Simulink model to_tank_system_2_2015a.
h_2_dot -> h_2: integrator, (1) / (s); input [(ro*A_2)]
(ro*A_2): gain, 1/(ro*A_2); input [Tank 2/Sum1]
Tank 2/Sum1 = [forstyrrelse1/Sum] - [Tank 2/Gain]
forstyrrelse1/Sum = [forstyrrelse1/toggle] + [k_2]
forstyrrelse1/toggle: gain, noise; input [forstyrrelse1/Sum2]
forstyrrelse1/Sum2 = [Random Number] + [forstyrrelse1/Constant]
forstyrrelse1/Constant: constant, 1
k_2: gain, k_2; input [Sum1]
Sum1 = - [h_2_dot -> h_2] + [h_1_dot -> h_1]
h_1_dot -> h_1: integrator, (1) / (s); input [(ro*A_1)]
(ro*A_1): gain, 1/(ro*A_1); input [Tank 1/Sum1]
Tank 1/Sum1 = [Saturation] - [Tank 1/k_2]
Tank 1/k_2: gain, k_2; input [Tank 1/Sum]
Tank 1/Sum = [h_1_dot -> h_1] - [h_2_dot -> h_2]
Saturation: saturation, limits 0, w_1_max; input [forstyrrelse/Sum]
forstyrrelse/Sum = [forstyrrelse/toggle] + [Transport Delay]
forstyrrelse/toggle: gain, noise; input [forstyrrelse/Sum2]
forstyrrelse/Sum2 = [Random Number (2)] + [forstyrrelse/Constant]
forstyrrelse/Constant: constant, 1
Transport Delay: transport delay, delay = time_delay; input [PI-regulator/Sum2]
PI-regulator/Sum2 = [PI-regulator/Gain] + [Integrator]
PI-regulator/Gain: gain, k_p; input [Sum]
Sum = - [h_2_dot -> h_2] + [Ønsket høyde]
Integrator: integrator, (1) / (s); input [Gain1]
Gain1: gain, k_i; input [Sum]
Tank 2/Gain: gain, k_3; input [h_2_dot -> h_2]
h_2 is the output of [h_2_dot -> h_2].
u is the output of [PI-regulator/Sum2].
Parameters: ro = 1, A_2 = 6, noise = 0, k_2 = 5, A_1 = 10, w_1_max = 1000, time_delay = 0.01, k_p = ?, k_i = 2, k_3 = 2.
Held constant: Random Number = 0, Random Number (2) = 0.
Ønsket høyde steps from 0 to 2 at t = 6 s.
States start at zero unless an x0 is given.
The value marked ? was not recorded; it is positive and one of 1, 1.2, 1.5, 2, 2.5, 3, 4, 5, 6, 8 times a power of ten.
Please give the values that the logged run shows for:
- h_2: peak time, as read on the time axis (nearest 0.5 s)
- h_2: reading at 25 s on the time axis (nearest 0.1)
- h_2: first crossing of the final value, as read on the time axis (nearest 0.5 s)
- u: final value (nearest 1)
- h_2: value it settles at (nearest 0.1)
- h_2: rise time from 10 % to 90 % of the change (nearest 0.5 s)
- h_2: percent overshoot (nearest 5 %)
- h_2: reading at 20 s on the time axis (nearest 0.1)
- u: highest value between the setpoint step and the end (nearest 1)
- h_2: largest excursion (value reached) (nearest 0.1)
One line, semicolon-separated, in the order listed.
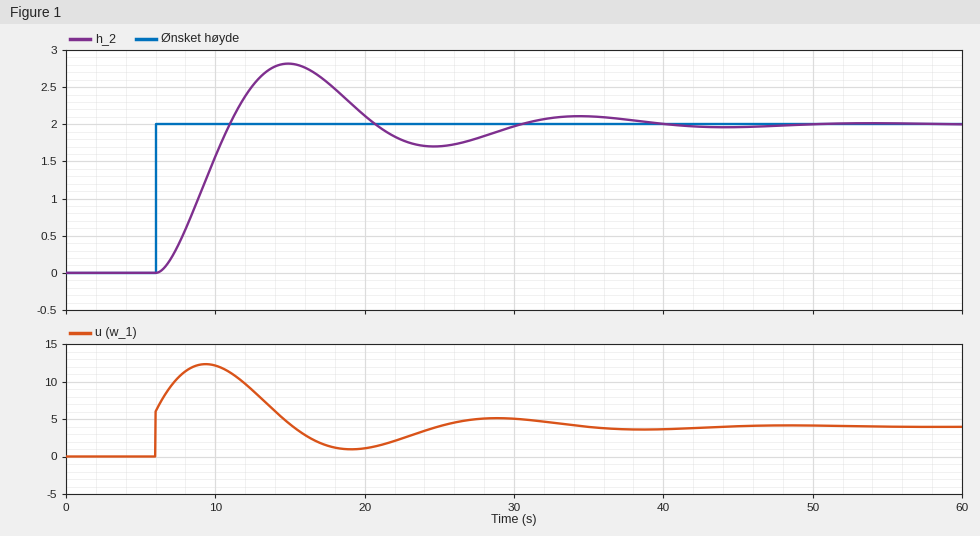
15.0 s; 1.7; 11.0 s; 4; 2.0; 3.5 s; 40 %; 2.1; 12; 2.8
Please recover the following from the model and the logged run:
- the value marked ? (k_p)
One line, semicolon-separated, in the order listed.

3
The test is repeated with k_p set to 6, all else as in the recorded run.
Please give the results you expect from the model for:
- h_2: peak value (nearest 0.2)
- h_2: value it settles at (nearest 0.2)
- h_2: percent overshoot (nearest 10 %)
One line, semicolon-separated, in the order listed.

2.4; 2.0; 20 %
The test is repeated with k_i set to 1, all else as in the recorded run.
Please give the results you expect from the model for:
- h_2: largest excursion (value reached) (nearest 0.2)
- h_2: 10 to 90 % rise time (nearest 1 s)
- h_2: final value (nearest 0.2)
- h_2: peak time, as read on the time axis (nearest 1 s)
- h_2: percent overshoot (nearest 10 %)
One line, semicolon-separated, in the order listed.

2.4; 5 s; 2.0; 18 s; 20 %
